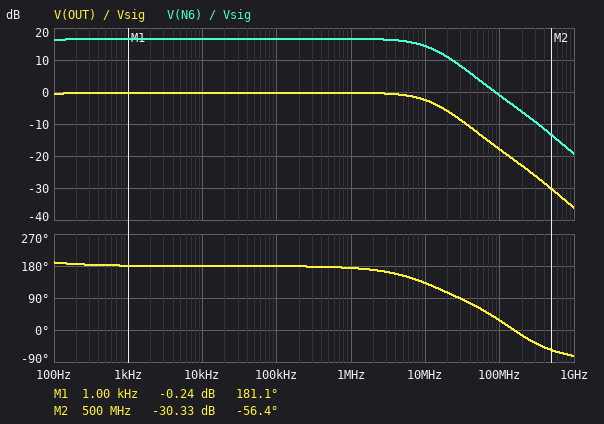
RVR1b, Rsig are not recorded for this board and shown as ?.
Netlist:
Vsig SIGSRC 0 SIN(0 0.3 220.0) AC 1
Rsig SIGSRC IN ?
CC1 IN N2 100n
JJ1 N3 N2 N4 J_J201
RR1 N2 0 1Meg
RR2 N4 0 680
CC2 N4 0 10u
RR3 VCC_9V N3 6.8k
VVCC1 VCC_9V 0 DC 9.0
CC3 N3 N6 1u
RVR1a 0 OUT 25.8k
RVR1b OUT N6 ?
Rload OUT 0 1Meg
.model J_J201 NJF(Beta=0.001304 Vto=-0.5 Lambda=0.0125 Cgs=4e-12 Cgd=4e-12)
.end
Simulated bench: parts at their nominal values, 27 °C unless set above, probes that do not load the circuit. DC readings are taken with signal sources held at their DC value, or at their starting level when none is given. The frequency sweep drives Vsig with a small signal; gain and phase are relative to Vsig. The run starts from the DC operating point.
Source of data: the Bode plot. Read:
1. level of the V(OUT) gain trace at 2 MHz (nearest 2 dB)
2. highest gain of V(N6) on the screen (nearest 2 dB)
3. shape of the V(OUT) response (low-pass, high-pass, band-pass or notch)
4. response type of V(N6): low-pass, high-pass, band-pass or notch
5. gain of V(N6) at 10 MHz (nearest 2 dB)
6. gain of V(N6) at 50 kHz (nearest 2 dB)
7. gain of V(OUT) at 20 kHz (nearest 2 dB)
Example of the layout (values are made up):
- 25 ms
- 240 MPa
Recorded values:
- 0 dB
- 16 dB
- low-pass
- low-pass
- 14 dB
- 16 dB
- 0 dB
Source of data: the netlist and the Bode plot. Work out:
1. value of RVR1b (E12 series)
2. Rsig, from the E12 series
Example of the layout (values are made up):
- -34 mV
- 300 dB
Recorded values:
- 150 kΩ
- 390 Ω
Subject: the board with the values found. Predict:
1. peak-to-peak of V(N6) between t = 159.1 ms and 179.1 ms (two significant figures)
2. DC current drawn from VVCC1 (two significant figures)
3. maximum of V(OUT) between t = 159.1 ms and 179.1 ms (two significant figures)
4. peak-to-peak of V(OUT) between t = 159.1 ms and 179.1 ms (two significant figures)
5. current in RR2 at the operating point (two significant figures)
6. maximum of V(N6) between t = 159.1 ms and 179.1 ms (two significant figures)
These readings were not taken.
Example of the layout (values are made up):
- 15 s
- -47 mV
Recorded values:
- 3.7 V
- 190 µA
- 200 mV
- 530 mV
- 190 µA
- 1.4 V
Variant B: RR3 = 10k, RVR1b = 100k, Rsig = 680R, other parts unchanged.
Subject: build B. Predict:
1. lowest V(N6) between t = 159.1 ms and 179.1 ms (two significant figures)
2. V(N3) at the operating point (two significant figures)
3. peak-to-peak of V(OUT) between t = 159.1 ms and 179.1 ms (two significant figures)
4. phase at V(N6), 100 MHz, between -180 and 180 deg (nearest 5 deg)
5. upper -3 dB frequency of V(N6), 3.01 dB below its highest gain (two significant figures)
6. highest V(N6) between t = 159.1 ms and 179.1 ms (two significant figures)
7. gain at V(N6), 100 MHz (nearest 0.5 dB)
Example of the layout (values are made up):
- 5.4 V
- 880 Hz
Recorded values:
- -3.2 V
- 7.1 V
- 1.0 V
- 15 deg
- 6.6 MHz
- 2.0 V
- -4.0 dB
